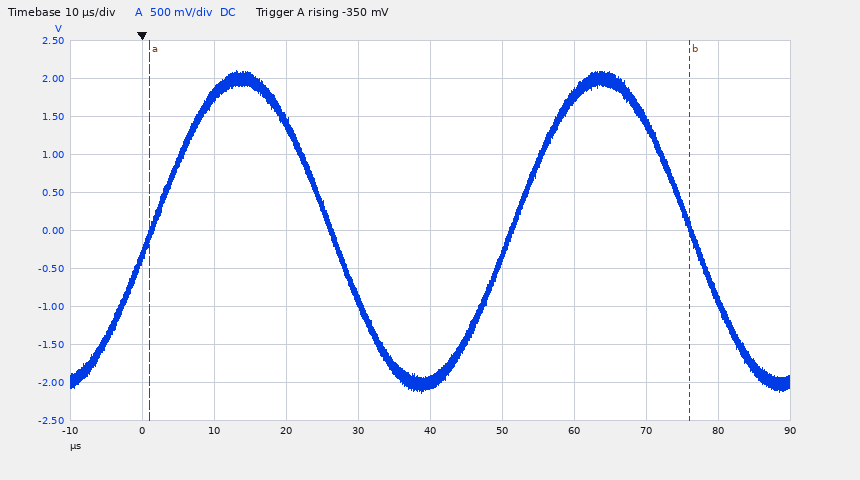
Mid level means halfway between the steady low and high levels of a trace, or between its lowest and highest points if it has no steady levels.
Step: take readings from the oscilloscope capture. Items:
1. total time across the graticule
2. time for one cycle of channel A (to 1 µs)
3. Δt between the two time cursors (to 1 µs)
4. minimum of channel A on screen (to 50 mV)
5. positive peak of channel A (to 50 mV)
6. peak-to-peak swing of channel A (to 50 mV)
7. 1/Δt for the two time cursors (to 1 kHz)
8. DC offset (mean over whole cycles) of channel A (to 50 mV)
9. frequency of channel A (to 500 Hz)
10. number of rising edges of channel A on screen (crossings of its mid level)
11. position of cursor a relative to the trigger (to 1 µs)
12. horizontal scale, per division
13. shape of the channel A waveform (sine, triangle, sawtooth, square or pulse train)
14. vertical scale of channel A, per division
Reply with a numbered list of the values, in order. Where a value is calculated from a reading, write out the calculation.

1. 100 µs
2. 50 µs
3. 75 µs
4. -2.15 V
5. 2.10 V
6. 2.10 V − (-2.15 V) = 4.25 V
7. 1 / 75 µs ≈ 13 kHz
8. (2.10 V + (-2.15 V)) / 2 ≈ 0 mV
9. 1 / 50 µs ≈ 20.0 kHz
10. 2
11. +1 µs
12. 10 µs
13. sine
14. 500 mV
